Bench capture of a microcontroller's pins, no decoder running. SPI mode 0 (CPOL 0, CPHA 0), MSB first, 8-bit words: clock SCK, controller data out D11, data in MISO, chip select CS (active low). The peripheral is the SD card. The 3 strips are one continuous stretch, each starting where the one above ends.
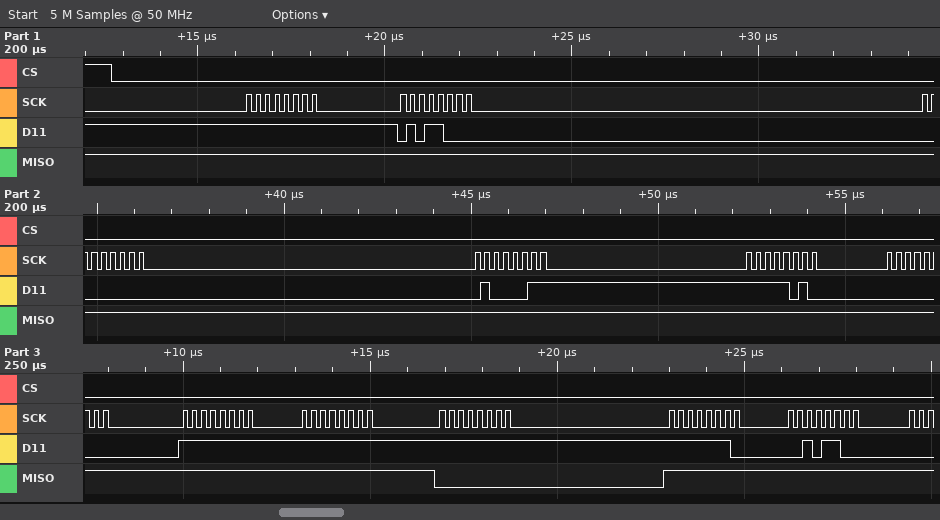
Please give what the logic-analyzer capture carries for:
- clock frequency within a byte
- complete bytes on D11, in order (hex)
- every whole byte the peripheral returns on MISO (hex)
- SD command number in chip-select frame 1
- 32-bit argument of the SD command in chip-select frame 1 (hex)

4 MHz
0xFF 0x58 0x00 0x43 0xFA 0x00 0xFF 0xFF 0xFF 0xFE 0x2C
0xFF 0xFF 0xFF 0xFF 0xFF 0xFF 0xFF 0xFF 0x00 0xFF 0xFF
CMD24
0x0043FA00
